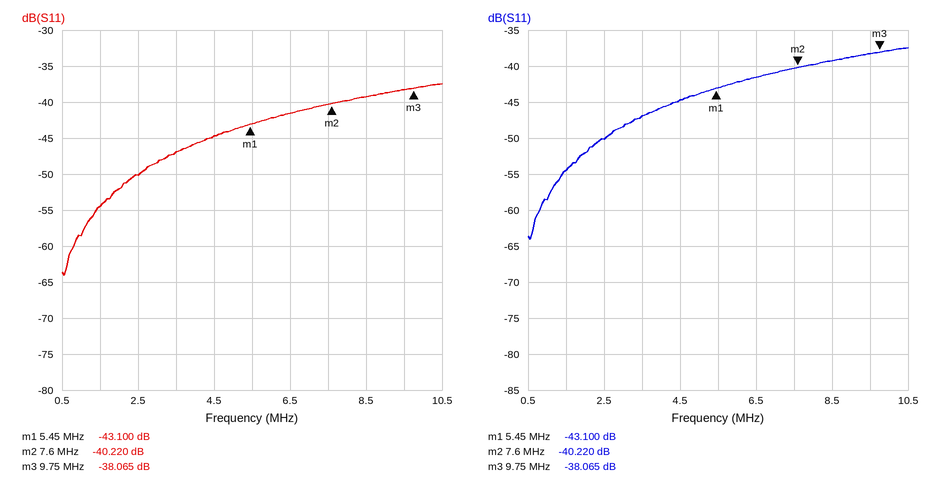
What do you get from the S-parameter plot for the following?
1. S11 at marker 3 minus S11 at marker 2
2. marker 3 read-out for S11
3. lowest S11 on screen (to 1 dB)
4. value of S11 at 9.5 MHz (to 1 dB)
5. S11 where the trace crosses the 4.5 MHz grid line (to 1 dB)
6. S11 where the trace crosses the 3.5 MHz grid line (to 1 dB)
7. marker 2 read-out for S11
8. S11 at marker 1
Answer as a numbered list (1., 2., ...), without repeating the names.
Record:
1. 2.155 dB
2. -38.065 dB
3. -64 dB
4. -38 dB
5. -45 dB
6. -47 dB
7. -40.220 dB
8. -43.100 dB
